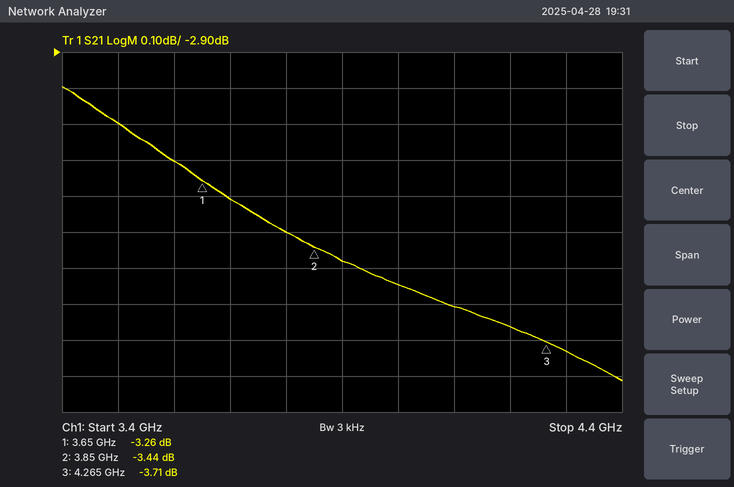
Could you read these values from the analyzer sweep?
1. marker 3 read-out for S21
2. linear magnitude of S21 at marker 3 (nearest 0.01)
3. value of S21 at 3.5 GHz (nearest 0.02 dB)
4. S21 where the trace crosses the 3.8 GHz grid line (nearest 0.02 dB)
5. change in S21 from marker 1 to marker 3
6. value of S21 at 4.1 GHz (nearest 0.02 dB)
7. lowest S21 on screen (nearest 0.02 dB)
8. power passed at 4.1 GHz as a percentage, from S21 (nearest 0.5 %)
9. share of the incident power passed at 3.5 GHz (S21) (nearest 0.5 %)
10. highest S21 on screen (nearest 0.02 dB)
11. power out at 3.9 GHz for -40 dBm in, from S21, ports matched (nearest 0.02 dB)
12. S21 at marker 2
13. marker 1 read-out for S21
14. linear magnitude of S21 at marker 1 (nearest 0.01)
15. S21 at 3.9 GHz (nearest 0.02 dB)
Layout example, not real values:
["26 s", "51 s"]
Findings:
["-3.71 dB", "0.65", "-3.10 dB", "-3.40 dB", "-0.45 dB", "-3.60 dB", "-3.82 dB", "43.5 %", "49.0 %", "-3.00 dB", "-43.48 dBm", "-3.44 dB", "-3.26 dB", "0.69", "-3.48 dB"]
